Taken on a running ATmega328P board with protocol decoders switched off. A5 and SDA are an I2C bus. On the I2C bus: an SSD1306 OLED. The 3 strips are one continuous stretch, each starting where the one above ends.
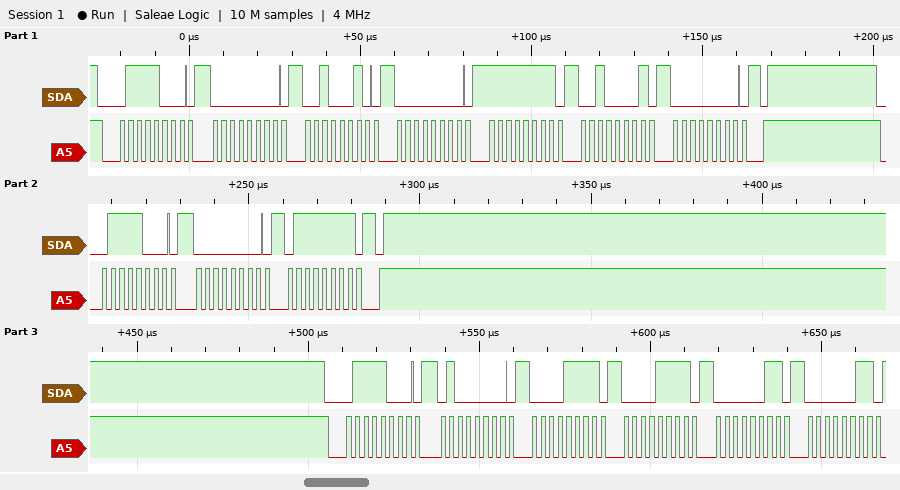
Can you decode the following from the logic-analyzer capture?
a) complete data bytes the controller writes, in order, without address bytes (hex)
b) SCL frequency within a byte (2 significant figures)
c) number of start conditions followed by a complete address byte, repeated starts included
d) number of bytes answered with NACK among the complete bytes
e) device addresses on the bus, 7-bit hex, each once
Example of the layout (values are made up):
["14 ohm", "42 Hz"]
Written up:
["00 22 00 FF 21 00 00 7F 40 0F 0F 03 03", "400 kHz", "3", "0", "0x3C"]
